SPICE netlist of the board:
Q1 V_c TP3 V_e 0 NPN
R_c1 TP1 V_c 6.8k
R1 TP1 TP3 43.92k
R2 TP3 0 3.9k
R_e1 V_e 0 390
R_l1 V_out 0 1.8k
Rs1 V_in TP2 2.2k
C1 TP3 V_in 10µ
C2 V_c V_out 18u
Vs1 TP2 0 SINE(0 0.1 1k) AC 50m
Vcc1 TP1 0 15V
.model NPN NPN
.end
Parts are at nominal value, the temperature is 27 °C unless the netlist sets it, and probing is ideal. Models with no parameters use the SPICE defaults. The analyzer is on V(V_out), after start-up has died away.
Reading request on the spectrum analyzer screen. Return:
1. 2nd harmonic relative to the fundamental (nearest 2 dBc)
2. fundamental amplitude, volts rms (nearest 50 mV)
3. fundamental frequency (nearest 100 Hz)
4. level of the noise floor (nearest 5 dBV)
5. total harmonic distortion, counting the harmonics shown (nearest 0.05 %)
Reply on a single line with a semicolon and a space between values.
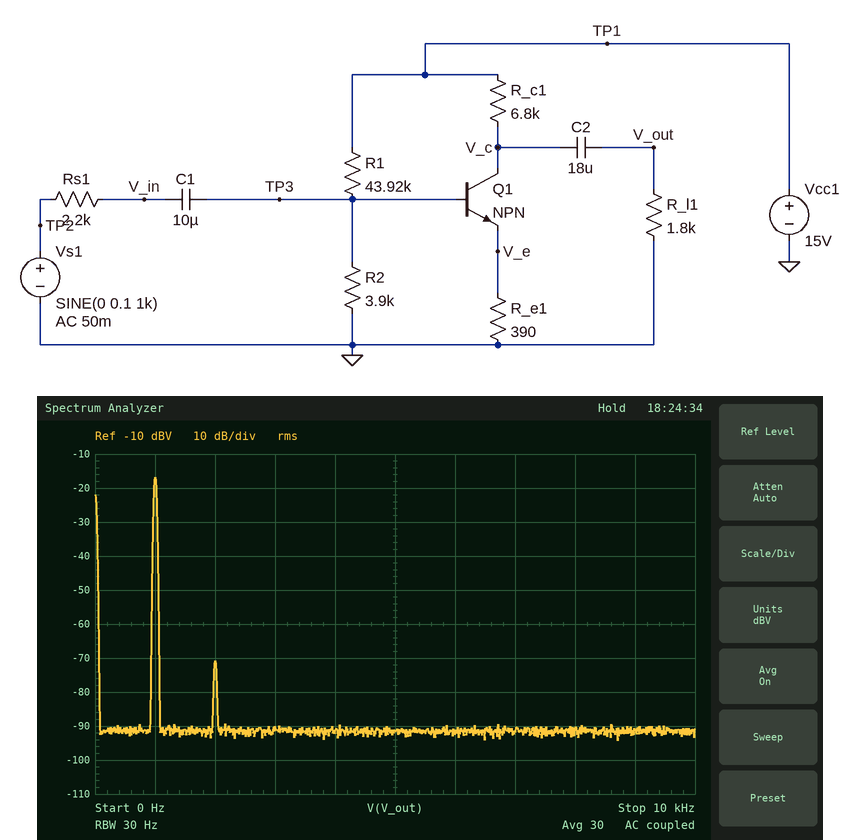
-54 dBc; 150 mV; 1.0 kHz; -90 dBV; 0.20 %
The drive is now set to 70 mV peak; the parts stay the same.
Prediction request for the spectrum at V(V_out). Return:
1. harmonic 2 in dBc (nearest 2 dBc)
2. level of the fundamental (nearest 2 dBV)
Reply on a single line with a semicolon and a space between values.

-58 dBc; -20 dBV
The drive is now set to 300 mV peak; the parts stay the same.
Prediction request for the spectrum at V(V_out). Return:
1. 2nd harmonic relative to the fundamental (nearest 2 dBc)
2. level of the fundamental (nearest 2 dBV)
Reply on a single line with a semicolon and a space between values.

-44 dBc; -8 dBV
